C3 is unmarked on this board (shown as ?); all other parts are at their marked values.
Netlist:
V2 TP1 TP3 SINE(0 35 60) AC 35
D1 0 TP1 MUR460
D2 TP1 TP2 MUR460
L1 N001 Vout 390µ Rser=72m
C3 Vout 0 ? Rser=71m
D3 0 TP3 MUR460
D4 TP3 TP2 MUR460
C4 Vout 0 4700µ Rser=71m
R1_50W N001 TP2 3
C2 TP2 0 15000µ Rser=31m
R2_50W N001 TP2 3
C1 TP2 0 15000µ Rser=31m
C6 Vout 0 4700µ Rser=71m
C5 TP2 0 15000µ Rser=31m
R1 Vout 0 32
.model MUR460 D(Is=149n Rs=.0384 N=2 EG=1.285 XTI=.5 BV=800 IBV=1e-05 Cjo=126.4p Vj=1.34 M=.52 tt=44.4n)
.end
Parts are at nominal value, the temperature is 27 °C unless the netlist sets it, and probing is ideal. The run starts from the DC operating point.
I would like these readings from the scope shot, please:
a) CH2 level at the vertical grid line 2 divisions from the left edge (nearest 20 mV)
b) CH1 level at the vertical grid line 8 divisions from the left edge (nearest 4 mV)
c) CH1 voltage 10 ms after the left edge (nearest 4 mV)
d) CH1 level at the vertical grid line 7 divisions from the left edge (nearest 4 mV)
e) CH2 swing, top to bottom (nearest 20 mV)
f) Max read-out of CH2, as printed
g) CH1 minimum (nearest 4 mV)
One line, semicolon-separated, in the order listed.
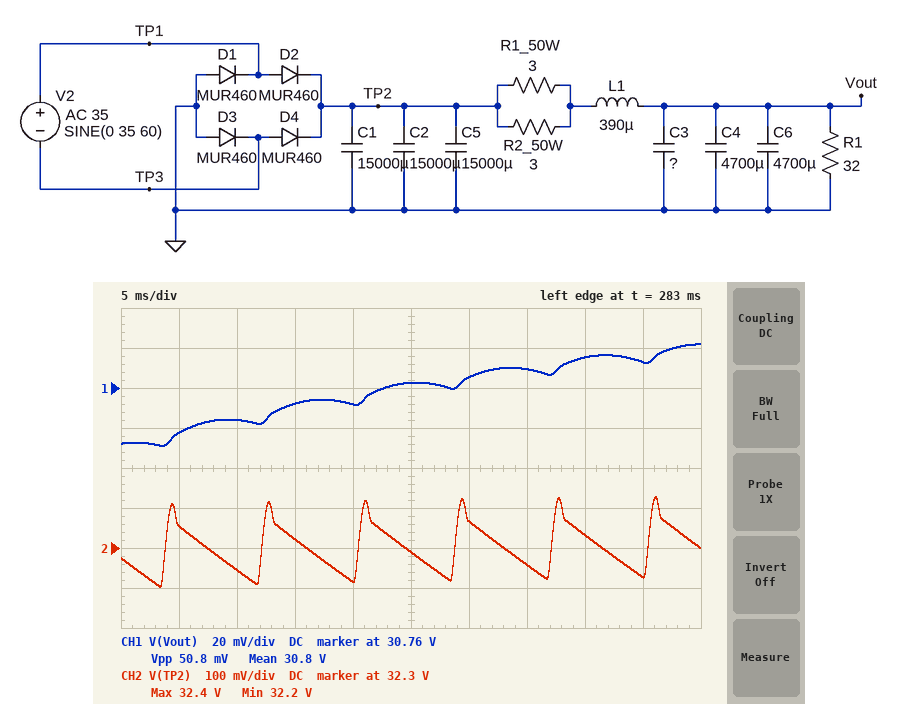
32.24 V; 30.776 V; 30.744 V; 30.768 V; 220 mV; 32.4 V; 30.732 V
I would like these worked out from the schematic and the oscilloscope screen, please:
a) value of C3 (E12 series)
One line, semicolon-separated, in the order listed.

10 mF
